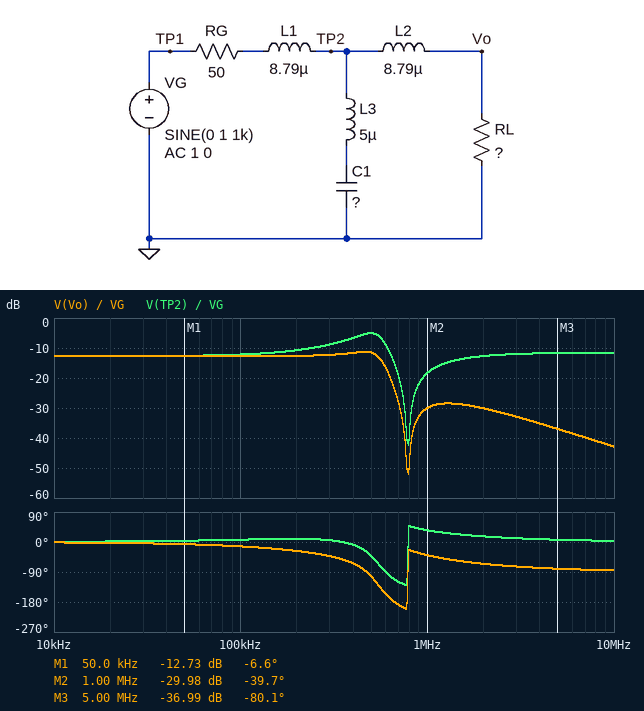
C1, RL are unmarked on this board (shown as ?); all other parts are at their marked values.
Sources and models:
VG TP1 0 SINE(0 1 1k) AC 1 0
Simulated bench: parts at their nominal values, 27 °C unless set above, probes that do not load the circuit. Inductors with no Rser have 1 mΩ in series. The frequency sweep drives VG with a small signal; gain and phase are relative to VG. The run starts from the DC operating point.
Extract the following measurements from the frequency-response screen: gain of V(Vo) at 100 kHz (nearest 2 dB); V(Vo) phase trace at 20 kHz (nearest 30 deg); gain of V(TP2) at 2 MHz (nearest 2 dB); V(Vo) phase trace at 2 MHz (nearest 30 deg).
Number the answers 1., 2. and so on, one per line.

1. -12 dB
2. 0 deg
3. -12 dB
4. -60 deg
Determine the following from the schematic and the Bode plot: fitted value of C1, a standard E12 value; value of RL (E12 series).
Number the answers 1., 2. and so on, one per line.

1. 8.2 nF
2. 15 Ω
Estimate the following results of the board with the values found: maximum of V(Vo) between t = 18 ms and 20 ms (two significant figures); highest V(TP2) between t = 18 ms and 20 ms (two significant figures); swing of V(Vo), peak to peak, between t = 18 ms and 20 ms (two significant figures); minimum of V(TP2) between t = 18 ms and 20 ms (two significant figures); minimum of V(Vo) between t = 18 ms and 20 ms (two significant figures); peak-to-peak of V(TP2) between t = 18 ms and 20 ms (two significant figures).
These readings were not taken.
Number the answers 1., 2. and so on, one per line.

1. 230 mV
2. 230 mV
3. 460 mV
4. -230 mV
5. -230 mV
6. 460 mV
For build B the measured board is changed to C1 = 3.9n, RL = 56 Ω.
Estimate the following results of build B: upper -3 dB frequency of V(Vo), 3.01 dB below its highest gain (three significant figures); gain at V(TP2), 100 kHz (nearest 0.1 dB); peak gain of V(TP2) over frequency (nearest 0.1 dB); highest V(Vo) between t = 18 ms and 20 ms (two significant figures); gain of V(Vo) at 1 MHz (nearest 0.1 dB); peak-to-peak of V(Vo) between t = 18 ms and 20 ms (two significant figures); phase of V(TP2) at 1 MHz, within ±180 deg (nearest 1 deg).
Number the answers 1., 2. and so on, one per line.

1. 813 kHz
2. -5.5 dB
3. -4.3 dB
4. 530 mV
5. -19.4 dB
6. 1.1 V
7. -126 deg
